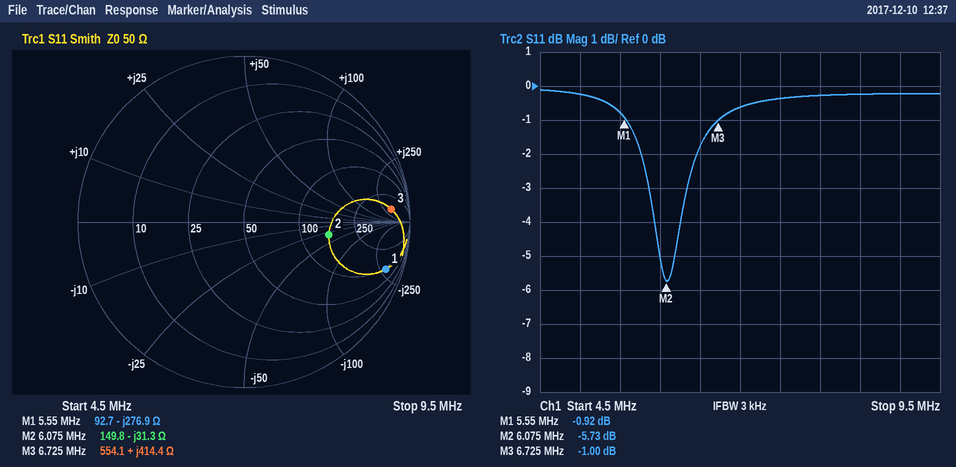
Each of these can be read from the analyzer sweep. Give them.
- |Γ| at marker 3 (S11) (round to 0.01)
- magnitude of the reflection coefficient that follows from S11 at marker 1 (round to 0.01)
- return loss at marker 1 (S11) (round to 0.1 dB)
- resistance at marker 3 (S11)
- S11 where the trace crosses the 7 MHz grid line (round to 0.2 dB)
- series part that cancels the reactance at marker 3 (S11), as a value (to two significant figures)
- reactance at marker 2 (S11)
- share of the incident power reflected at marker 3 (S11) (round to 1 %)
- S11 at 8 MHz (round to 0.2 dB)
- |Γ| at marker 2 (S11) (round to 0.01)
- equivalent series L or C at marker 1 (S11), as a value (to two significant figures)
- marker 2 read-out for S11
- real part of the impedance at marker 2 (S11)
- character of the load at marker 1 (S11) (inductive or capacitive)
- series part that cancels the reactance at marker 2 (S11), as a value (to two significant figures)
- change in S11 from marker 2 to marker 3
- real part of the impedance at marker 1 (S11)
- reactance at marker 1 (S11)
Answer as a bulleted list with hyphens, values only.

- 0.89
- 0.90
- 0.9 dB
- 554.1 Ω
- -0.6 dB
- 57 pF
- -31.3 Ω
- 79 %
- -0.2 dB
- 0.52
- 100 pF
- -5.73 dB
- 149.8 Ω
- capacitive
- 820 nH
- 4.73 dB
- 92.7 Ω
- -276.9 Ω
